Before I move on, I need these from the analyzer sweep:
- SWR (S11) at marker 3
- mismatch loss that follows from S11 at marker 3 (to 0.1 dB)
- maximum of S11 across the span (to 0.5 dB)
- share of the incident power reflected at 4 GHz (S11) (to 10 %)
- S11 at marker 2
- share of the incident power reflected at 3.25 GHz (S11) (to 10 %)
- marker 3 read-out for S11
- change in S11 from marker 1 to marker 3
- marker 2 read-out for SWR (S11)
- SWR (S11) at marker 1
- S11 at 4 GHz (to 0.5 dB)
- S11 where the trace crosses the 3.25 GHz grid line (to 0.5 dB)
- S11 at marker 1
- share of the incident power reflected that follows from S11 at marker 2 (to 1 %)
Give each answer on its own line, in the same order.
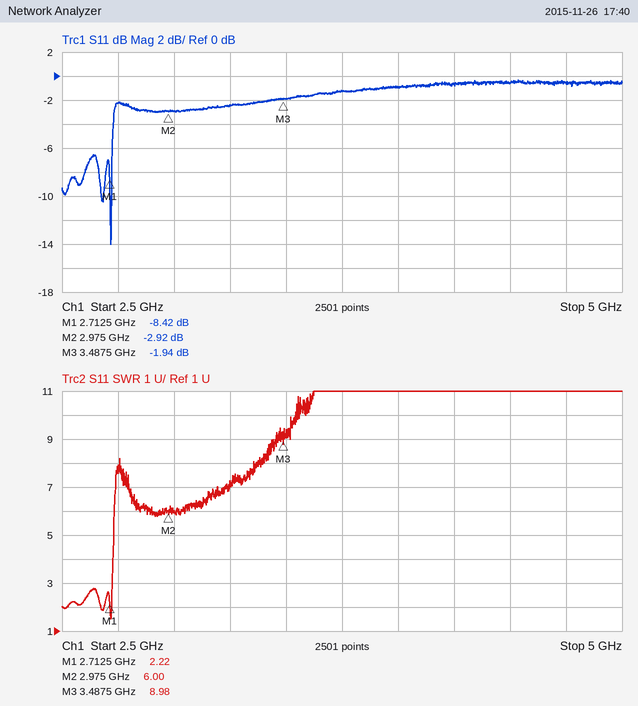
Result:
8.98
4.4 dB
-0.5 dB
80 %
-2.92 dB
60 %
-1.94 dB
6.48 dB
6.00
2.22
-1.0 dB
-2.5 dB
-8.42 dB
51 %
